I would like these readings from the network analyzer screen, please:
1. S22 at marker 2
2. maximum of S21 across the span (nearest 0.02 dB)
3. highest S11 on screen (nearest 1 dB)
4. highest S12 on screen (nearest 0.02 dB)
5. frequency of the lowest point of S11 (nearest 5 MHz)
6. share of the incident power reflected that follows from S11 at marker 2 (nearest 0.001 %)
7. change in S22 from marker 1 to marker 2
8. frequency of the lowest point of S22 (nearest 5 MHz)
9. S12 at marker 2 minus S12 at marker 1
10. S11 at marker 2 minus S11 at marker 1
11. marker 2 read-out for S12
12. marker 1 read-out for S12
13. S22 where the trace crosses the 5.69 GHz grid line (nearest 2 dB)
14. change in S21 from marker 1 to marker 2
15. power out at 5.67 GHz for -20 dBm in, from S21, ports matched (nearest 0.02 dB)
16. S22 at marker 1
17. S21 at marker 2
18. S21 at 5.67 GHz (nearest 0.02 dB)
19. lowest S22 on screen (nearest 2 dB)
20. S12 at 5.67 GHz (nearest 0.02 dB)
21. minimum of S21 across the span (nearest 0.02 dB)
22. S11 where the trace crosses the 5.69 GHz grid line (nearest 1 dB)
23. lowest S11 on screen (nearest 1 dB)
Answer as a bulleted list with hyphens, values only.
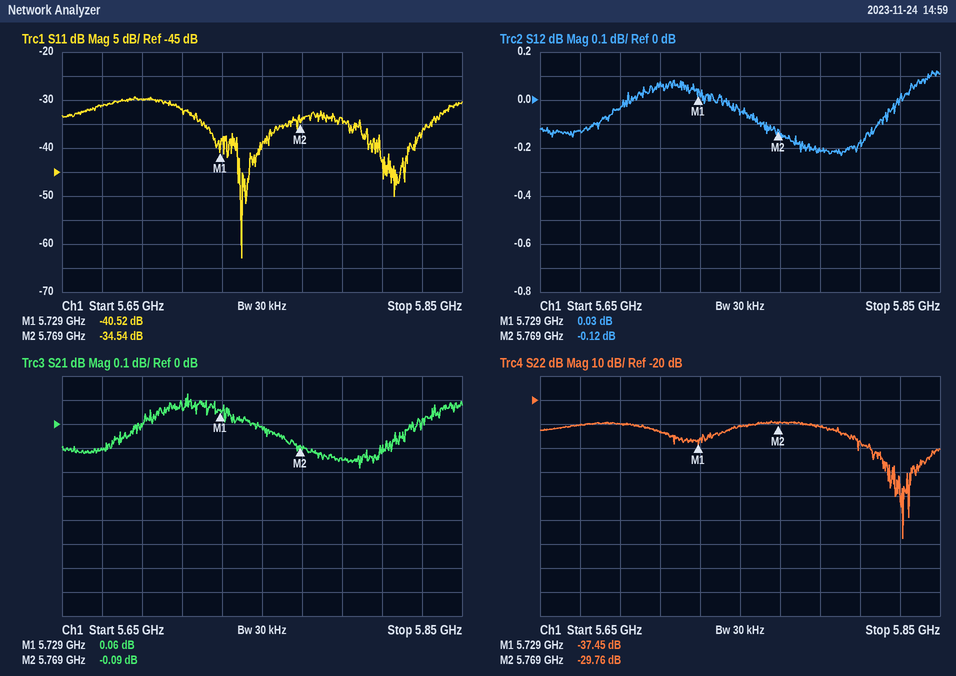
- -29.76 dB
- 0.12 dB
- -29 dB
- 0.12 dB
- 5.740 GHz
- 0.035 %
- 7.69 dB
- 5.830 GHz
- -0.15 dB
- 5.98 dB
- -0.12 dB
- 0.03 dB
- -30 dB
- -0.15 dB
- -20.10 dBm
- -37.45 dB
- -0.09 dB
- -0.10 dB
- -78 dB
- -0.12 dB
- -0.18 dB
- -30 dB
- -63 dB
